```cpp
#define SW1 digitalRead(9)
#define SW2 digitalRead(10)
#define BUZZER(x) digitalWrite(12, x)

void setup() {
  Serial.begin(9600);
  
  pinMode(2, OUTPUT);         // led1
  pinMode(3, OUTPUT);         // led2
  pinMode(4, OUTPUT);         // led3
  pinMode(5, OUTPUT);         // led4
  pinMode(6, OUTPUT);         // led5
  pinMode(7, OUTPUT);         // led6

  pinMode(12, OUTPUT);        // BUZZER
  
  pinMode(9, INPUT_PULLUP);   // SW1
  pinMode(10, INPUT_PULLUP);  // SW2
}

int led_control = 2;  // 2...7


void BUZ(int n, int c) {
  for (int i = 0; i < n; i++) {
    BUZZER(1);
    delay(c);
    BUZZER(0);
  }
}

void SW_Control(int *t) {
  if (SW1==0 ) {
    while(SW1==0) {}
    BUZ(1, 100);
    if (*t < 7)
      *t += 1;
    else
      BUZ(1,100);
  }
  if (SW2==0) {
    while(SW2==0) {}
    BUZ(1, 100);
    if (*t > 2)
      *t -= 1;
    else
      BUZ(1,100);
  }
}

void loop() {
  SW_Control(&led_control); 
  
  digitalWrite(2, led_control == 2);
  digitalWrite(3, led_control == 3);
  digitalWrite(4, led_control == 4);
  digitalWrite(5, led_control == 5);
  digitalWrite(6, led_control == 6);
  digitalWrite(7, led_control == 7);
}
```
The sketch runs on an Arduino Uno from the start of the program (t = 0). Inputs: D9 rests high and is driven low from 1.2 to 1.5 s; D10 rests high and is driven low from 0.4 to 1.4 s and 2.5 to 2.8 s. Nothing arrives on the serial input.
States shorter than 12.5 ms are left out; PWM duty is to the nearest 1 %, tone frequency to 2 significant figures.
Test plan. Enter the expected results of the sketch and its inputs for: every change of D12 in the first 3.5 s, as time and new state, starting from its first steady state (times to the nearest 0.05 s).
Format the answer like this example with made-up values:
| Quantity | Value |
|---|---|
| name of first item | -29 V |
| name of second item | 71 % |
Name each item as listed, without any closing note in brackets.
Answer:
| Quantity | Value |
|---|---|
| every change of D12 in the first 3.5 s, as time and new state, starting from its first steady state | 0 s low; 1.4 s high; 1.6 s low; 2.8 s high; 3 s low |
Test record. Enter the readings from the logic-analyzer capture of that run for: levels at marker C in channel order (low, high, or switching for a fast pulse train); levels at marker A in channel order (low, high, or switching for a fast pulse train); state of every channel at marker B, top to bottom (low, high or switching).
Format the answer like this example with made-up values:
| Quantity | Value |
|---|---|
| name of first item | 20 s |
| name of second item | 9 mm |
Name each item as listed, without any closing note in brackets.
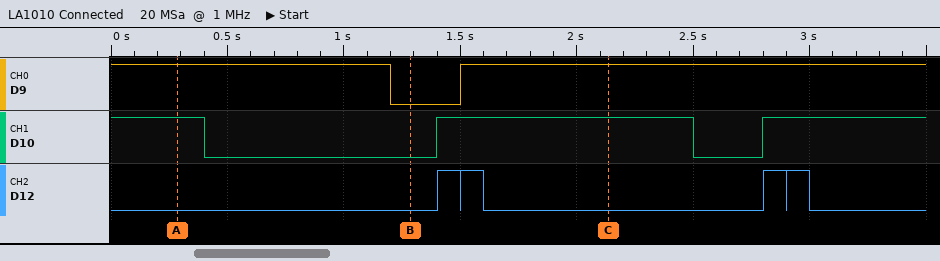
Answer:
| Quantity | Value |
|---|---|
| levels at marker C in channel order | D9 high, D10 high, D12 low |
| levels at marker A in channel order | D9 high, D10 high, D12 low |
| state of every channel at marker B, top to bottom | D9 low, D10 low, D12 low |
